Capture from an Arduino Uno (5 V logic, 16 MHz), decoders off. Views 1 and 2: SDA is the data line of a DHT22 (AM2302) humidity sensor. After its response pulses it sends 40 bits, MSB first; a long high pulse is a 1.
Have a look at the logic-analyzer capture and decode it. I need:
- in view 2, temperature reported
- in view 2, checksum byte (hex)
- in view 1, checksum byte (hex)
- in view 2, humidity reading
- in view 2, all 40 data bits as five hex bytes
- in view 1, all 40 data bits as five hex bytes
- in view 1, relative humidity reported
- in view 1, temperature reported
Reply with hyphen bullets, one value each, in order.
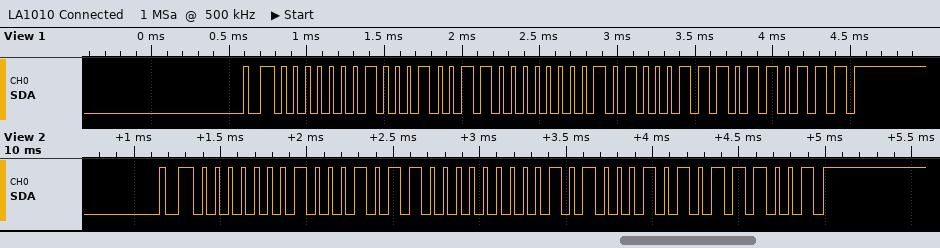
- 16.2 °C
- 0xB9
- 0xB7
- 27.8 %
- 01 16 00 A2 B9
- 01 13 00 A3 B7
- 27.5 %
- 16.3 °C
